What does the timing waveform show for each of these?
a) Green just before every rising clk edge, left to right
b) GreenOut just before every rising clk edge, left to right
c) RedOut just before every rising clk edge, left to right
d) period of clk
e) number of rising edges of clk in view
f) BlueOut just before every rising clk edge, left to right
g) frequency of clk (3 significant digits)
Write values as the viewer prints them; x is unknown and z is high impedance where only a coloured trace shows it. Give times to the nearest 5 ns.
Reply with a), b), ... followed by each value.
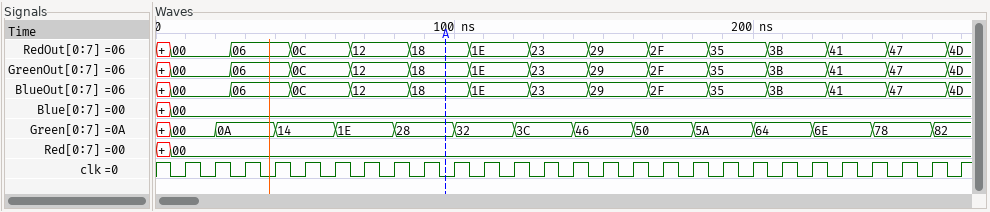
a) 00, 00, 0A, 0A, 14, 14, 1E, 1E, 28, 28, 32, 32, 3C, 3C, 46, 46, 50, 50, 5A, 5A, 64, 64, 6E, 6E, 78, 78, 82
b) 00, 00, 06, 06, 0C, 0C, 12, 12, 18, 18, 1E, 1E, 23, 23, 29, 29, 2F, 2F, 35, 35, 3B, 3B, 41, 41, 47, 47, 4D
c) 00, 00, 06, 06, 0C, 0C, 12, 12, 18, 18, 1E, 1E, 23, 23, 29, 29, 2F, 2F, 35, 35, 3B, 3B, 41, 41, 47, 47, 4D
d) 10 ns
e) 27
f) 00, 00, 06, 06, 0C, 0C, 12, 12, 18, 18, 1E, 1E, 23, 23, 29, 29, 2F, 2F, 35, 35, 3B, 3B, 41, 41, 47, 47, 4D
g) 100 MHz
